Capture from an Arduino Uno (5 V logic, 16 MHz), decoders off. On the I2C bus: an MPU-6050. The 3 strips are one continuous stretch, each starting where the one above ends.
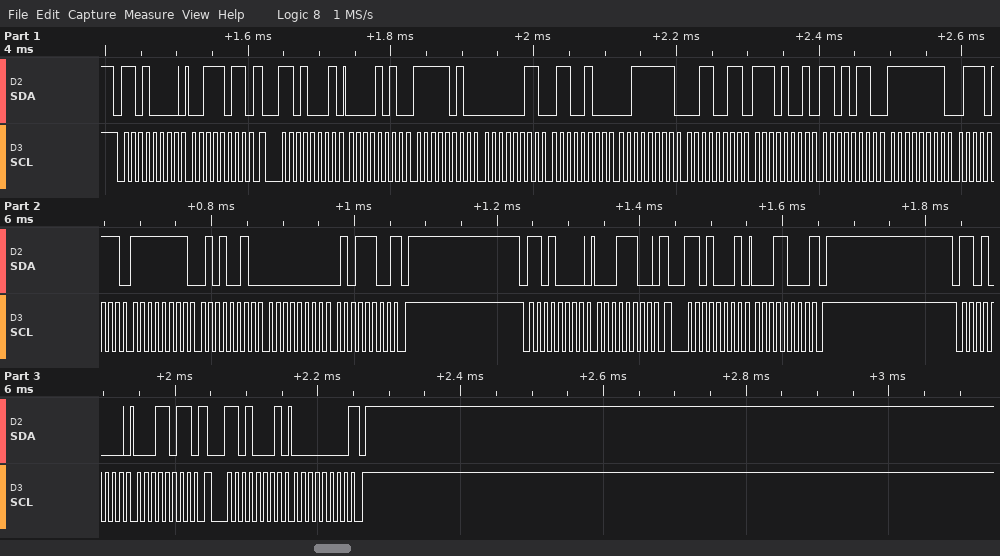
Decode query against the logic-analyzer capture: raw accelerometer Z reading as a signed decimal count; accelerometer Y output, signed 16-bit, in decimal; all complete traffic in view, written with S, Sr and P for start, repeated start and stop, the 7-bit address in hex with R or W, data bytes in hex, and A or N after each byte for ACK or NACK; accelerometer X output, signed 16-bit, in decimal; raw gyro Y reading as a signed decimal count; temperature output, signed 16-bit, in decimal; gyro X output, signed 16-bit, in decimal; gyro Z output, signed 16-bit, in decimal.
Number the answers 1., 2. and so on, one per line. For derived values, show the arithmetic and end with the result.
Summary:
1. 0x3F33 = 16179
2. 0x0364 = 868
3. S 68W A 3B A Sr 68R A 0A A FA A 03 A 64 A 3F A 33 A E9 A D6 A FF A 77 A FF A 52 A 00 A 5C N P S 68W A 1C A Sr 68R A 18 N P S 68W A 1B A Sr 68R A 00 N P
4. 0x0AFA = 2810
5. 0xFF52 = -174
6. 0xE9D6 = -5674
7. 0xFF77 = -137
8. 0x005C = 92
